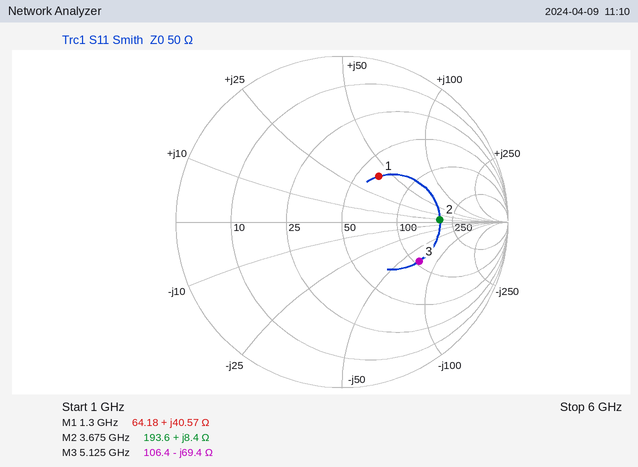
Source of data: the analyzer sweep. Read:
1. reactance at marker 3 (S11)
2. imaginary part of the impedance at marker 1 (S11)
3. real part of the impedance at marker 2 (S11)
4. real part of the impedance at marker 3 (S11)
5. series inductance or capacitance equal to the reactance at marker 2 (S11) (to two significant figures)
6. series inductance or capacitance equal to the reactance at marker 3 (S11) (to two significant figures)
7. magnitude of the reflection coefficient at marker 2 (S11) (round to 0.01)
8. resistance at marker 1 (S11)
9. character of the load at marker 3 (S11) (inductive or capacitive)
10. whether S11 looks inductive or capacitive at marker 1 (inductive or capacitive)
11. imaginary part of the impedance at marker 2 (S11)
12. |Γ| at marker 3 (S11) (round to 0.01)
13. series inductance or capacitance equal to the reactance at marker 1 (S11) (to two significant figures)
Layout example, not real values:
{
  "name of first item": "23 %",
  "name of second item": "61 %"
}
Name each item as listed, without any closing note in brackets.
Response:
{
  "reactance at marker 3": "-69.4 Ω",
  "imaginary part of the impedance at marker 1": "+40.57 Ω",
  "real part of the impedance at marker 2": "193.6 Ω",
  "real part of the impedance at marker 3": "106.4 Ω",
  "series inductance or capacitance equal to the reactance at marker 2 (S11)": "360 pH",
  "series inductance or capacitance equal to the reactance at marker 3 (S11)": "450 fF",
  "magnitude of the reflection coefficient at marker 2 (S11)": "0.59",
  "resistance at marker 1": "64.18 Ω",
  "character of the load at marker 3 (S11)": "capacitive",
  "whether S11 looks inductive or capacitive at marker 1": "inductive",
  "imaginary part of the impedance at marker 2": "+8.4 Ω",
  "|Γ| at marker 3 (S11)": "0.52",
  "series inductance or capacitance equal to the reactance at marker 1 (S11)": "5.0 nH"
}
